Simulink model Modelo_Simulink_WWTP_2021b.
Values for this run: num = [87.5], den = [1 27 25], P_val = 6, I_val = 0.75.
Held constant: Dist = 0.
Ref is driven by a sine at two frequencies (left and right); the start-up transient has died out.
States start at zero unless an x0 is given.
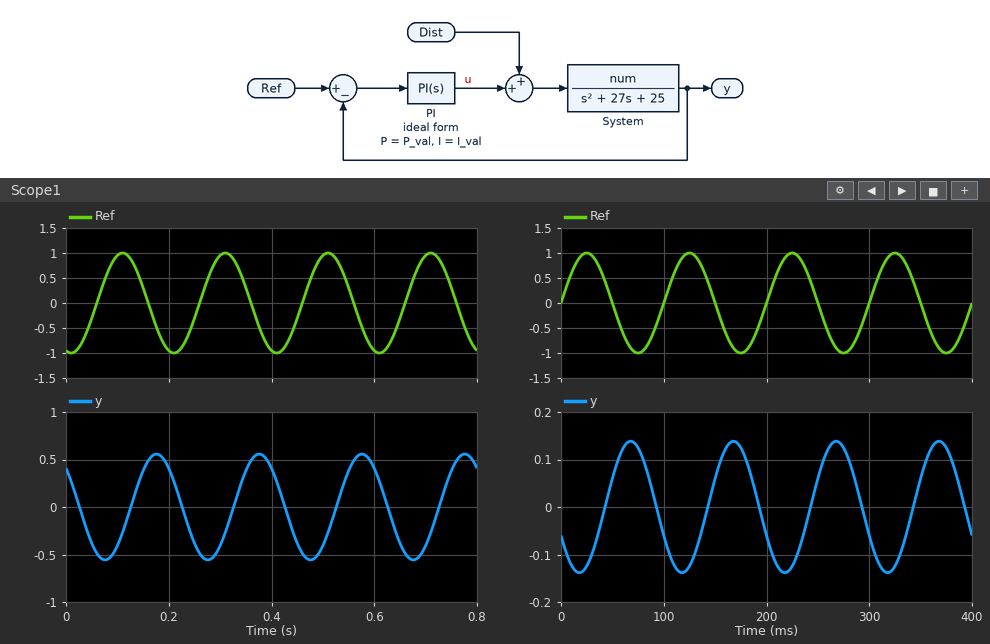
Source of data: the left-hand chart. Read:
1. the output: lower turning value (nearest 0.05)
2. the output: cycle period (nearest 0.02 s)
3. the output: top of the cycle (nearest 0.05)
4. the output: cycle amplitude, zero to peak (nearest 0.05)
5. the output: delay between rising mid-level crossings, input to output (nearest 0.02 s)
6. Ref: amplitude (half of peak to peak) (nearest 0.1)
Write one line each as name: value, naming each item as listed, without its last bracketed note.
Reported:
the output: lower turning value: -0.55
the output: cycle period: 0.20 s
the output: top of the cycle: 0.55
the output: cycle amplitude, zero to peak: 0.55
the output: delay between rising mid-level crossings, input to output: 0.06 s
Ref: amplitude (half of peak to peak): 1.0
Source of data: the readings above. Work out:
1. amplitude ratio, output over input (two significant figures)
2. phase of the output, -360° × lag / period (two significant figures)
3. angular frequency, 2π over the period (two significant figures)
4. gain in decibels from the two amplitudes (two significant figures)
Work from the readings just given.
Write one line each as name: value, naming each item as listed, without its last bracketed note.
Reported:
amplitude ratio, output over input: 0.55
phase of the output, -360° × lag / period: -110°
angular frequency, 2π over the period: 31 rad/s
gain in decibels from the two amplitudes: -5.2 dB
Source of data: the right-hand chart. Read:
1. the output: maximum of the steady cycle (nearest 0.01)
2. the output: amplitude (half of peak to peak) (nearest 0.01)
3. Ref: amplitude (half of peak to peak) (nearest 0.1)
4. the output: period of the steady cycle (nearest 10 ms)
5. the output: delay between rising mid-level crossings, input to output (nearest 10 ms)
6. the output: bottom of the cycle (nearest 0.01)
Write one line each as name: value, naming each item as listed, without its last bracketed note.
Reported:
the output: maximum of the steady cycle: 0.14
the output: amplitude (half of peak to peak): 0.14
Ref: amplitude (half of peak to peak): 1.0
the output: period of the steady cycle: 100 ms
the output: delay between rising mid-level crossings, input to output: 40 ms
the output: bottom of the cycle: -0.14
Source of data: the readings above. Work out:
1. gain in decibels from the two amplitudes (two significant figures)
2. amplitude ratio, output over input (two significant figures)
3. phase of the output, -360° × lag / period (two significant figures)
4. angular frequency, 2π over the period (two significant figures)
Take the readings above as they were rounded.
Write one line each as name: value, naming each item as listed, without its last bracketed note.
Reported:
gain in decibels from the two amplitudes: -17 dB
amplitude ratio, output over input: 0.14
phase of the output, -360° × lag / period: -140°
angular frequency, 2π over the period: 0.063 rad/ms
